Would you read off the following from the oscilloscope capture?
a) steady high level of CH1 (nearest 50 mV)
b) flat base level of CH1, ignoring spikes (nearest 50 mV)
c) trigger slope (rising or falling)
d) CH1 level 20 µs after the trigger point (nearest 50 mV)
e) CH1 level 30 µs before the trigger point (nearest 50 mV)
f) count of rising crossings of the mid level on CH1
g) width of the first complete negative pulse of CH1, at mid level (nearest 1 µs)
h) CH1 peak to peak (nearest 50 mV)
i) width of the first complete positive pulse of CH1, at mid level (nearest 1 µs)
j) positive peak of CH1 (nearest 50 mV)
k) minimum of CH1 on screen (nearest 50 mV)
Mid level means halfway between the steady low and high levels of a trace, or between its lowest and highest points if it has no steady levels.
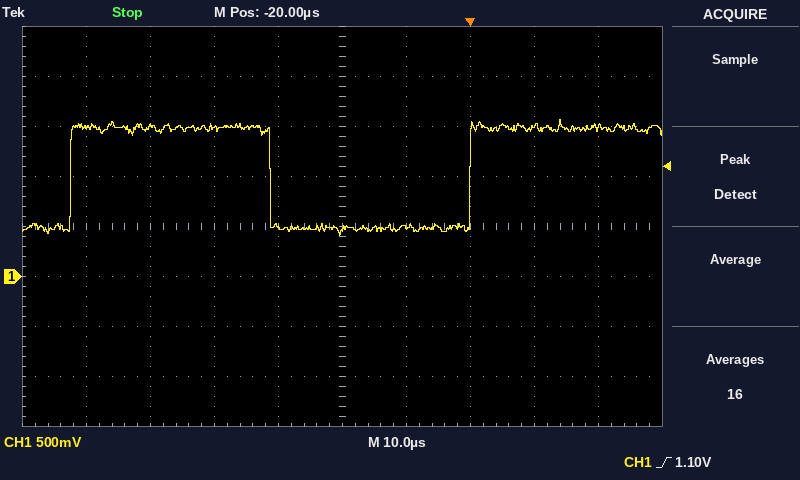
1.50 V
500 mV
rising
1.50 V
500 mV
2
31 µs
1.15 V
31 µs
1.55 V
400 mV
